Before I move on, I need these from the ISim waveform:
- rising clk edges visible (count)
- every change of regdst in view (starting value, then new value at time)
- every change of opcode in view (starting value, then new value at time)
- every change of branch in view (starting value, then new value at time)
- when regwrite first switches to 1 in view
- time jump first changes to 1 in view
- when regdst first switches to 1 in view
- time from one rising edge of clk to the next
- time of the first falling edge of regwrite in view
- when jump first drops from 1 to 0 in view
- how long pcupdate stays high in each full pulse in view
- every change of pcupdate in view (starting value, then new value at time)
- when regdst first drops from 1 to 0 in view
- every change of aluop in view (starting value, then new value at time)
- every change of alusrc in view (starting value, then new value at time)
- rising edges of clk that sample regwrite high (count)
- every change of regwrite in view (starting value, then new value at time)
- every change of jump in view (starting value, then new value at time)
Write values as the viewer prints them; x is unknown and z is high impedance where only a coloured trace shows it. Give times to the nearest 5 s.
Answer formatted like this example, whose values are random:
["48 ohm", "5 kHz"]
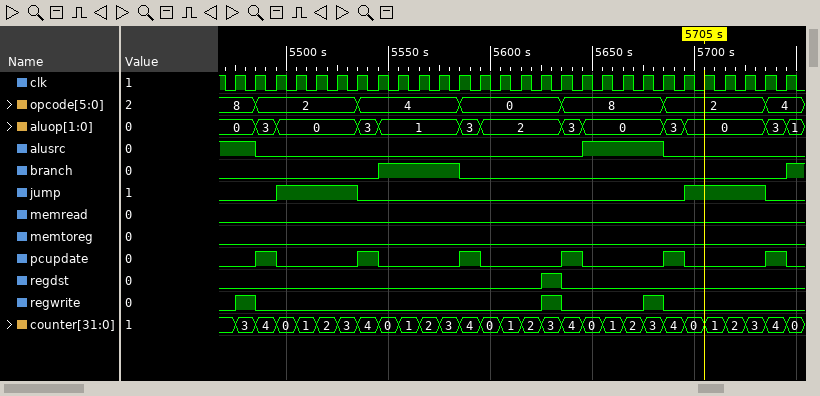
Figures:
["28", "0, 1 at 5625 s, 0 at 5635 s", "8, 2 at 5485 s, 4 at 5535 s, 0 at 5585 s, 8 at 5635 s, 2 at 5685 s, 4 at 5735 s", "0, 1 at 5545 s, 0 at 5585 s, 1 at 5745 s", "5475 s", "5495 s", "5625 s", "10 s", "5485 s", "5535 s", "10 s, 10 s, 10 s, 10 s, 10 s, 10 s", "0, 1 at 5485 s, 0 at 5495 s, 1 at 5535 s, 0 at 5545 s, 1 at 5585 s, 0 at 5595 s, 1 at 5635 s, 0 at 5645 s, 1 at 5685 s, 0 at 5695 s, 1 at 5735 s, 0 at 5745 s", "5635 s", "0, 3 at 5485 s, 0 at 5495 s, 3 at 5535 s, 1 at 5545 s, 3 at 5585 s, 2 at 5595 s, 3 at 5635 s, 0 at 5645 s, 3 at 5685 s, 0 at 5695 s, 3 at 5735 s, 1 at 5745 s", "1, 0 at 5485 s, 1 at 5645 s, 0 at 5685 s", "3", "0, 1 at 5475 s, 0 at 5485 s, 1 at 5625 s, 0 at 5635 s, 1 at 5675 s, 0 at 5685 s", "0, 1 at 5495 s, 0 at 5535 s, 1 at 5695 s, 0 at 5735 s"]
